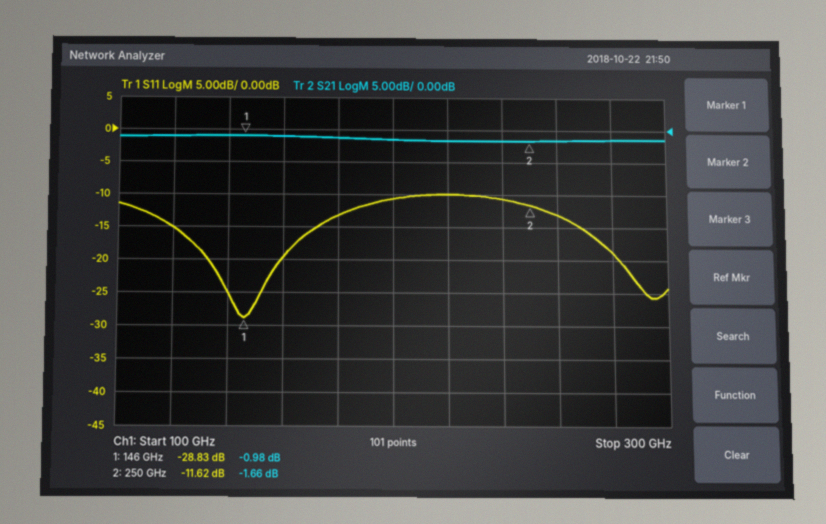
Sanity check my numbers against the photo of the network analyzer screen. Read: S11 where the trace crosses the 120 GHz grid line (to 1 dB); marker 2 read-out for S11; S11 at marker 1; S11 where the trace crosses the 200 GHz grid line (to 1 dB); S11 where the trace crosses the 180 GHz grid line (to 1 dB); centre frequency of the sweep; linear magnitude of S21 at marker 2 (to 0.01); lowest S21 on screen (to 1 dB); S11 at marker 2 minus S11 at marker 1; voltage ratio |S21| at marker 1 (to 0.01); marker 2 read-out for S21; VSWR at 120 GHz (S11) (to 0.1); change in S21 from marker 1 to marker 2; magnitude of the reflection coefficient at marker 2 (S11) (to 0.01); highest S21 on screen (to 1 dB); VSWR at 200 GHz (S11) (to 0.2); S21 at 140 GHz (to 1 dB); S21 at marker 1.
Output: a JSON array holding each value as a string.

["-15 dB", "-11.62 dB", "-28.83 dB", "-11 dB", "-13 dB", "200 GHz", "0.83", "-2 dB", "17.21 dB", "0.89", "-1.66 dB", "1.4", "-0.68 dB", "0.26", "-1 dB", "1.8", "-1 dB", "-0.98 dB"]
